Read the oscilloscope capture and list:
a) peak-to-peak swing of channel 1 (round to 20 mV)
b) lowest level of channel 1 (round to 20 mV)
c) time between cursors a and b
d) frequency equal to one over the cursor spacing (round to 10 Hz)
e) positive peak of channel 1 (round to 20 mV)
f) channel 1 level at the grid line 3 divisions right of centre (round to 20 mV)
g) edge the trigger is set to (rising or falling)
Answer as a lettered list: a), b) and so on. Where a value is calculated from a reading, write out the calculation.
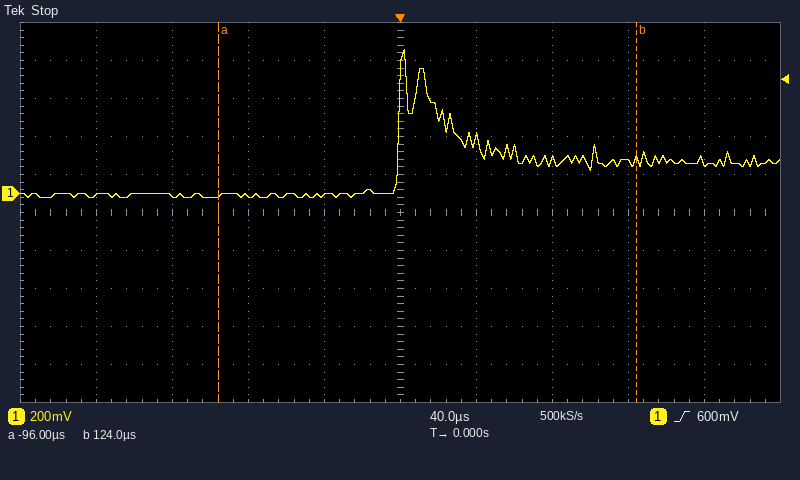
a) 760 mV − (-20 mV) = 780 mV
b) -20 mV
c) 124 µs − (-96 µs) = 220 µs
d) 1 / 220 µs ≈ 4.55 kHz
e) 760 mV
f) 160 mV
g) rising
